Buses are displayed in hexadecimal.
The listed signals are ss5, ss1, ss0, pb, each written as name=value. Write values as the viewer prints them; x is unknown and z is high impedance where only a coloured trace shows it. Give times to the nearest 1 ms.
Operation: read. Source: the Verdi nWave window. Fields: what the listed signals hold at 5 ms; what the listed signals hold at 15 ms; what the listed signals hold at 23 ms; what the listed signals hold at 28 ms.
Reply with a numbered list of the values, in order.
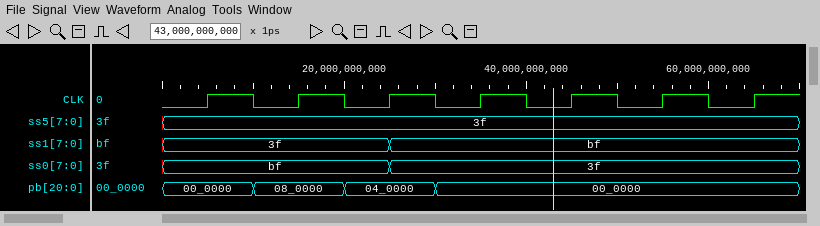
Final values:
1. ss5=3f, ss1=3f, ss0=bf, pb=00_0000
2. ss5=3f, ss1=3f, ss0=bf, pb=08_0000
3. ss5=3f, ss1=3f, ss0=bf, pb=04_0000
4. ss5=3f, ss1=bf, ss0=3f, pb=04_0000
